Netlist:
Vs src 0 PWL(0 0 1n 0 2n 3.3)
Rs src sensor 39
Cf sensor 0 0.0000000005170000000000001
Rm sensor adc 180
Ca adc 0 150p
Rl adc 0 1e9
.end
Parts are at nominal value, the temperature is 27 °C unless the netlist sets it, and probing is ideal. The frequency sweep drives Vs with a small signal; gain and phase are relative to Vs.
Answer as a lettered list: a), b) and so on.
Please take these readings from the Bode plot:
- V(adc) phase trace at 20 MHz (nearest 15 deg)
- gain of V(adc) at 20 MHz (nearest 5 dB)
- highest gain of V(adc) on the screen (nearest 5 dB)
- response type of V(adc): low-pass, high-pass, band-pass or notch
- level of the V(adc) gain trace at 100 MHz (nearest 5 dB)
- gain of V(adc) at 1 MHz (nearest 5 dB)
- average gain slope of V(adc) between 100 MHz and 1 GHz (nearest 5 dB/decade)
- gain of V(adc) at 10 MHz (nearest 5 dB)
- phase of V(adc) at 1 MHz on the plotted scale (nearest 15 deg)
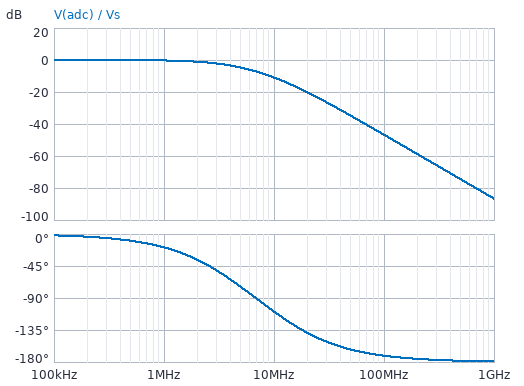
a) -135 deg
b) -20 dB
c) 0 dB
d) low-pass
e) -45 dB
f) 0 dB
g) -40 dB/decade
h) -10 dB
i) -15 deg
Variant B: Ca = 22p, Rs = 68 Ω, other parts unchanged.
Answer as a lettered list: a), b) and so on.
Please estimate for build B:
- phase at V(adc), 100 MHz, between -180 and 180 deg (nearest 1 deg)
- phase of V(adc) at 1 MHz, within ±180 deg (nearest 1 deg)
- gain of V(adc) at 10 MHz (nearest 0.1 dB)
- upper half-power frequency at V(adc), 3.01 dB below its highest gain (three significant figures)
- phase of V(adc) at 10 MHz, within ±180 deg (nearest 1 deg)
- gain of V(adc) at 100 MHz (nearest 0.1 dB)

a) -155 deg
b) -14 deg
c) -8.3 dB
d) 4.28 MHz
e) -80 deg
f) -35.5 dB
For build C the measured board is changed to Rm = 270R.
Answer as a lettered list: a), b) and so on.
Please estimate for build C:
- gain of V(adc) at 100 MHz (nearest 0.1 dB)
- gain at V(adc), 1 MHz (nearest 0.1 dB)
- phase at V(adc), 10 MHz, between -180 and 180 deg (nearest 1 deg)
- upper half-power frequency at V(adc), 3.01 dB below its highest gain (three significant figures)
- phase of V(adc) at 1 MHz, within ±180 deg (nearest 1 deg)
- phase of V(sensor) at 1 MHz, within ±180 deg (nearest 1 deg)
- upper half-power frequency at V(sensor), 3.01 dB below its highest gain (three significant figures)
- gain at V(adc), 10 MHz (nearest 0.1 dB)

a) -50.2 dB
b) -0.5 dB
c) -118 deg
d) 2.90 MHz
e) -23 deg
f) -9 deg
g) 6.46 MHz
h) -13.5 dB
